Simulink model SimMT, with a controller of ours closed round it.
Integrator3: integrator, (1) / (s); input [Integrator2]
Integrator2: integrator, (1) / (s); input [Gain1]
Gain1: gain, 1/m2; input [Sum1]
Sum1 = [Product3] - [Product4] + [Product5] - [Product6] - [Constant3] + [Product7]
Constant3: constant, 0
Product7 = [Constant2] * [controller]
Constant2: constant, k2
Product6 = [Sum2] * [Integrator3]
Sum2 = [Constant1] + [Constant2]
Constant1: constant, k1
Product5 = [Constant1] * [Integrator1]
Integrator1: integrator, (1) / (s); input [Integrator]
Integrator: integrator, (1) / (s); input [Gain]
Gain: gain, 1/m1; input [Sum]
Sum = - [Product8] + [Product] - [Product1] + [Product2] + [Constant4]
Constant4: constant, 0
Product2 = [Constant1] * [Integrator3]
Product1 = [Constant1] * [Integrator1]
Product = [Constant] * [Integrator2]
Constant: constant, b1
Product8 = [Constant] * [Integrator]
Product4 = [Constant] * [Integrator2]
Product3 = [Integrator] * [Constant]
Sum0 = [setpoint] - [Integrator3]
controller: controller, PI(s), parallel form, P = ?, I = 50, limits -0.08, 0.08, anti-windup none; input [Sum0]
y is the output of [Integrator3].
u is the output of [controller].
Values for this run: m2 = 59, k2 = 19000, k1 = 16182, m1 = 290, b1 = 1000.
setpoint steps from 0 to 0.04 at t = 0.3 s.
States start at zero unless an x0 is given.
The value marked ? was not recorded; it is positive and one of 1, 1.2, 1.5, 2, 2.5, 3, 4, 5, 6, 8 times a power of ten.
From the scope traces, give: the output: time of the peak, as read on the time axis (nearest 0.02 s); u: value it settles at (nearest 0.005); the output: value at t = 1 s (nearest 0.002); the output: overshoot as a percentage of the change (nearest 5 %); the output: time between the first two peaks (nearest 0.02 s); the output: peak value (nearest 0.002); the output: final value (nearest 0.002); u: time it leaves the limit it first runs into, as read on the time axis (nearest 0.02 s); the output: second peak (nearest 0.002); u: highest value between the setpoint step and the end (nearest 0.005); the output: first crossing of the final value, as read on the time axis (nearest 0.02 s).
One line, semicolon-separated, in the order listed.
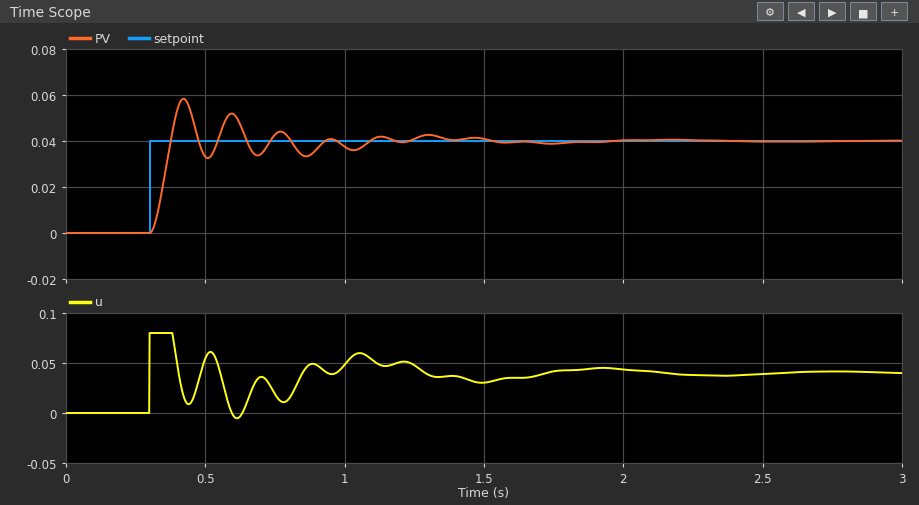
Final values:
0.42 s; 0.040; 0.038; 45 %; 0.18 s; 0.058; 0.040; 0.38 s; 0.052; 0.080; 0.38 s
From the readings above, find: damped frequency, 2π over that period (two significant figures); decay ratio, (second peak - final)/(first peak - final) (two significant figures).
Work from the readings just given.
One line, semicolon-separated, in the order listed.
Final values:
35 rad/s; 0.67
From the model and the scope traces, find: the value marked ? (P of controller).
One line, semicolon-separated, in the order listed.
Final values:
2.5
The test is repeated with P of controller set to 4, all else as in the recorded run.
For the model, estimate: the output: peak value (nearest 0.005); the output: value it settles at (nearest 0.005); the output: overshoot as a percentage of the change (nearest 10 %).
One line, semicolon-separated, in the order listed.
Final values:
0.055; 0.040; 40 %
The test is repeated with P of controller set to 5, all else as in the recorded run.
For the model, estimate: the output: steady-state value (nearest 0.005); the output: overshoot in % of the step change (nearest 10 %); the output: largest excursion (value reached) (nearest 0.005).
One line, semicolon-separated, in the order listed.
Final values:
0.040; 40 %; 0.055
